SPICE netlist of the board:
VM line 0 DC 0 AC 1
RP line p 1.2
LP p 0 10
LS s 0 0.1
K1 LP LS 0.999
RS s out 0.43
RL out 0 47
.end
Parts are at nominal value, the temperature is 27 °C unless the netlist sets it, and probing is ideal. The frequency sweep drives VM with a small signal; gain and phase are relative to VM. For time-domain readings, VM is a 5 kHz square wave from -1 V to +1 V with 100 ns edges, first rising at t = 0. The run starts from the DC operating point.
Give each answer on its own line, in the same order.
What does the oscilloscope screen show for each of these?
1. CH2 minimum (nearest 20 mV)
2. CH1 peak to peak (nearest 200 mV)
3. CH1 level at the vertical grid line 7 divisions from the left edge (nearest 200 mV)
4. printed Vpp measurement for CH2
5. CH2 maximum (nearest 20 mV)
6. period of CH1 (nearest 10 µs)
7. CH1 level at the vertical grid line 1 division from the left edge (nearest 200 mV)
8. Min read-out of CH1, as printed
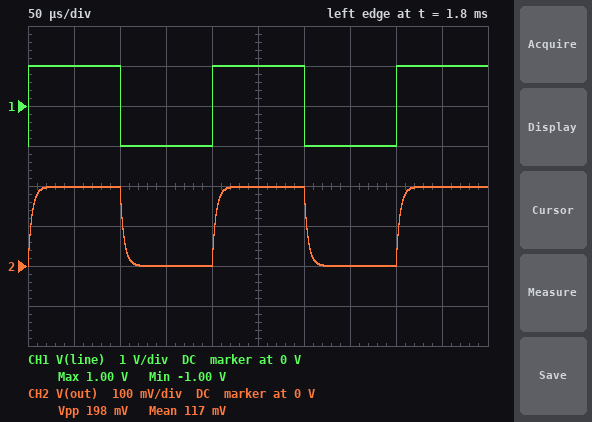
0 V
2.0 V
-1.0 V
198 mV
200 mV
200 µs
1.0 V
-1.00 V
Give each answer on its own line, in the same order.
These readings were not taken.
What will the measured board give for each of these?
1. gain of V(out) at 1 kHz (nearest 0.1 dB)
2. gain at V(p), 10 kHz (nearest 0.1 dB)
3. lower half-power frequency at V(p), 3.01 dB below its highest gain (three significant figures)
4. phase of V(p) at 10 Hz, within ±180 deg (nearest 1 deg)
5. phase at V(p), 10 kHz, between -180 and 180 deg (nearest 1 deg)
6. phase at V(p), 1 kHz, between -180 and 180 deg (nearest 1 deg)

-20.1 dB
0 dB
19.1 mHz
0 deg
0 deg
0 deg
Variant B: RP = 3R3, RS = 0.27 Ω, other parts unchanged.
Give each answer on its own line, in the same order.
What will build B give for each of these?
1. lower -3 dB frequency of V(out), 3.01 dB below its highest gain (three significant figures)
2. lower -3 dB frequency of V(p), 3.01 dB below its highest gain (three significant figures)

52.5 mHz
52.6 mHz
